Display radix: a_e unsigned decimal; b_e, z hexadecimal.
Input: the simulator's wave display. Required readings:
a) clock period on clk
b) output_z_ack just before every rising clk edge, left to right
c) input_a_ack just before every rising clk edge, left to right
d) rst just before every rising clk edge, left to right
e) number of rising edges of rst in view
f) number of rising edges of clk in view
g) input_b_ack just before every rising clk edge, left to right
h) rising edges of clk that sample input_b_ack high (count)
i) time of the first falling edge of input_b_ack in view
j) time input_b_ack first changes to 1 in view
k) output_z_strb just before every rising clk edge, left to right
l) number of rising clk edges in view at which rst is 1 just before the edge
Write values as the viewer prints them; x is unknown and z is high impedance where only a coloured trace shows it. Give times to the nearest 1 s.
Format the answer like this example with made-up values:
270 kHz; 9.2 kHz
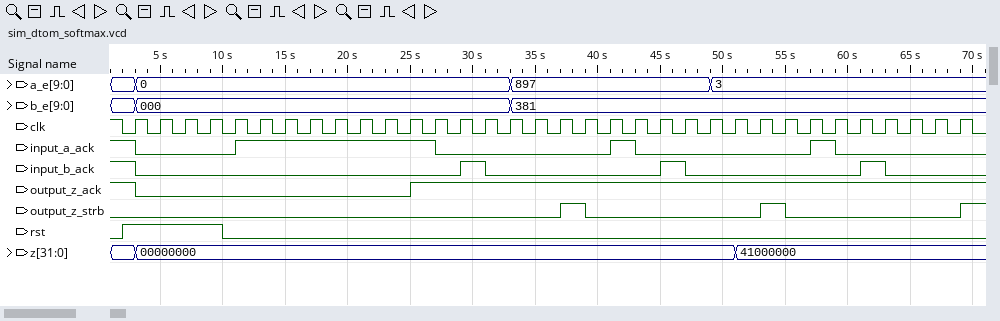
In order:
2 s; 1 0 0 0 0 0 0 0 0 0 0 0 1 1 1 1 1 1 1 1 1 1 1 1 1 1 1 1 1 1 1 1 1 1; 1 0 0 0 0 1 1 1 1 1 1 1 1 0 0 0 0 0 0 0 1 0 0 0 0 0 0 0 1 0 0 0 0 0; 1 1 1 1 0 0 0 0 0 0 0 0 0 0 0 0 0 0 0 0 0 0 0 0 0 0 0 0 0 0 0 0 0 0; 1; 34; 1 0 0 0 0 0 0 0 0 0 0 0 0 0 1 0 0 0 0 0 0 0 1 0 0 0 0 0 0 0 1 0 0 0; 4; 3 s; 29 s; 0 0 0 0 0 0 0 0 0 0 0 0 0 0 0 0 0 0 1 0 0 0 0 0 0 0 1 0 0 0 0 0 0 0; 4
